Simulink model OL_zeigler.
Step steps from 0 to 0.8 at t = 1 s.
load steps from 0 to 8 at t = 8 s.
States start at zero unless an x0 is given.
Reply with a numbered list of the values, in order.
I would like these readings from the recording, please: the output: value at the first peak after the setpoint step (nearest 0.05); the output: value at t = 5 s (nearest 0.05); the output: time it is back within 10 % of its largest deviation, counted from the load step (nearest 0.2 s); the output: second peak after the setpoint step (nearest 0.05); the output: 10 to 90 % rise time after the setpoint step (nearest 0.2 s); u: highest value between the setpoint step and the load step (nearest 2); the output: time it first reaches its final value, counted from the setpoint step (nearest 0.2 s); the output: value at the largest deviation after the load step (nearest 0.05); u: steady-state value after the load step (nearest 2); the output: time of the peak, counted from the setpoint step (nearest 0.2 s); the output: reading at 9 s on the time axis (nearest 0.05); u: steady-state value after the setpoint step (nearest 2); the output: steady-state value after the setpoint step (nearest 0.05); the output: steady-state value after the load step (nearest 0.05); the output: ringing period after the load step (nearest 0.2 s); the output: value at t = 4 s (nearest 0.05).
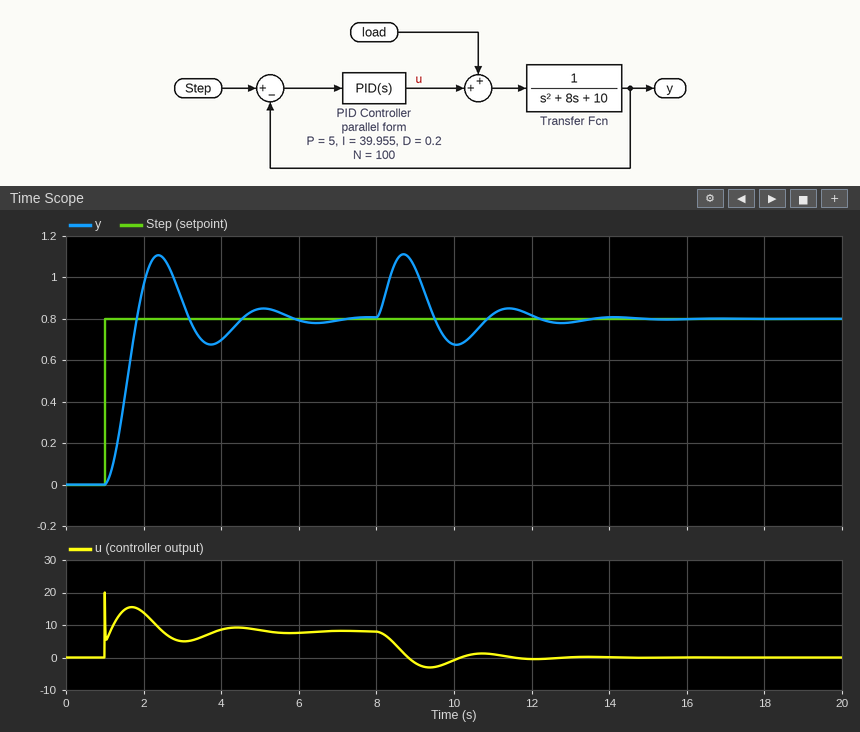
1. 1.10
2. 0.85
3. 3.8 s
4. 0.85
5. 0.6 s
6. 20
7. 0.8 s
8. 1.10
9. 0
10. 1.4 s
11. 1.05
12. 8
13. 0.80
14. 0.80
15. 2.8 s
16. 0.70
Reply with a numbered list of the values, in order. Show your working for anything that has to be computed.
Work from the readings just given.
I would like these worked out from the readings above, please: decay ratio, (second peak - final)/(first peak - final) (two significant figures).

1. (0.85 - 0.8) / (1.1 - 0.8) = 0.17
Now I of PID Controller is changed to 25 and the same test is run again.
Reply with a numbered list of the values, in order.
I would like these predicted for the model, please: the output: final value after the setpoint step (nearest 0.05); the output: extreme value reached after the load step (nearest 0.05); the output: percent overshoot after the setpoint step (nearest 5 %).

1. 0.80
2. 1.15
3. 20 %
